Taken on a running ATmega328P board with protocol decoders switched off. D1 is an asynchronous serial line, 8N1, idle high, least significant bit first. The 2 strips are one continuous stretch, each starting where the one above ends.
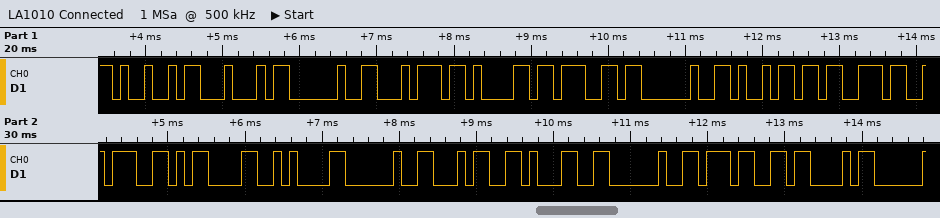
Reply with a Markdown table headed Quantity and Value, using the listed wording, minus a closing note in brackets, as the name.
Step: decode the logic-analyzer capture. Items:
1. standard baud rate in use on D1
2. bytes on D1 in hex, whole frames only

| Quantity | Value |
|---|---|
| standard baud rate in use on D1 | 9600 baud |
| bytes on D1 in hex, whole frames only | 49 44 20 74 61 67 20 69 73 3A 0D 0A 20 34 31 20 37 43 |
